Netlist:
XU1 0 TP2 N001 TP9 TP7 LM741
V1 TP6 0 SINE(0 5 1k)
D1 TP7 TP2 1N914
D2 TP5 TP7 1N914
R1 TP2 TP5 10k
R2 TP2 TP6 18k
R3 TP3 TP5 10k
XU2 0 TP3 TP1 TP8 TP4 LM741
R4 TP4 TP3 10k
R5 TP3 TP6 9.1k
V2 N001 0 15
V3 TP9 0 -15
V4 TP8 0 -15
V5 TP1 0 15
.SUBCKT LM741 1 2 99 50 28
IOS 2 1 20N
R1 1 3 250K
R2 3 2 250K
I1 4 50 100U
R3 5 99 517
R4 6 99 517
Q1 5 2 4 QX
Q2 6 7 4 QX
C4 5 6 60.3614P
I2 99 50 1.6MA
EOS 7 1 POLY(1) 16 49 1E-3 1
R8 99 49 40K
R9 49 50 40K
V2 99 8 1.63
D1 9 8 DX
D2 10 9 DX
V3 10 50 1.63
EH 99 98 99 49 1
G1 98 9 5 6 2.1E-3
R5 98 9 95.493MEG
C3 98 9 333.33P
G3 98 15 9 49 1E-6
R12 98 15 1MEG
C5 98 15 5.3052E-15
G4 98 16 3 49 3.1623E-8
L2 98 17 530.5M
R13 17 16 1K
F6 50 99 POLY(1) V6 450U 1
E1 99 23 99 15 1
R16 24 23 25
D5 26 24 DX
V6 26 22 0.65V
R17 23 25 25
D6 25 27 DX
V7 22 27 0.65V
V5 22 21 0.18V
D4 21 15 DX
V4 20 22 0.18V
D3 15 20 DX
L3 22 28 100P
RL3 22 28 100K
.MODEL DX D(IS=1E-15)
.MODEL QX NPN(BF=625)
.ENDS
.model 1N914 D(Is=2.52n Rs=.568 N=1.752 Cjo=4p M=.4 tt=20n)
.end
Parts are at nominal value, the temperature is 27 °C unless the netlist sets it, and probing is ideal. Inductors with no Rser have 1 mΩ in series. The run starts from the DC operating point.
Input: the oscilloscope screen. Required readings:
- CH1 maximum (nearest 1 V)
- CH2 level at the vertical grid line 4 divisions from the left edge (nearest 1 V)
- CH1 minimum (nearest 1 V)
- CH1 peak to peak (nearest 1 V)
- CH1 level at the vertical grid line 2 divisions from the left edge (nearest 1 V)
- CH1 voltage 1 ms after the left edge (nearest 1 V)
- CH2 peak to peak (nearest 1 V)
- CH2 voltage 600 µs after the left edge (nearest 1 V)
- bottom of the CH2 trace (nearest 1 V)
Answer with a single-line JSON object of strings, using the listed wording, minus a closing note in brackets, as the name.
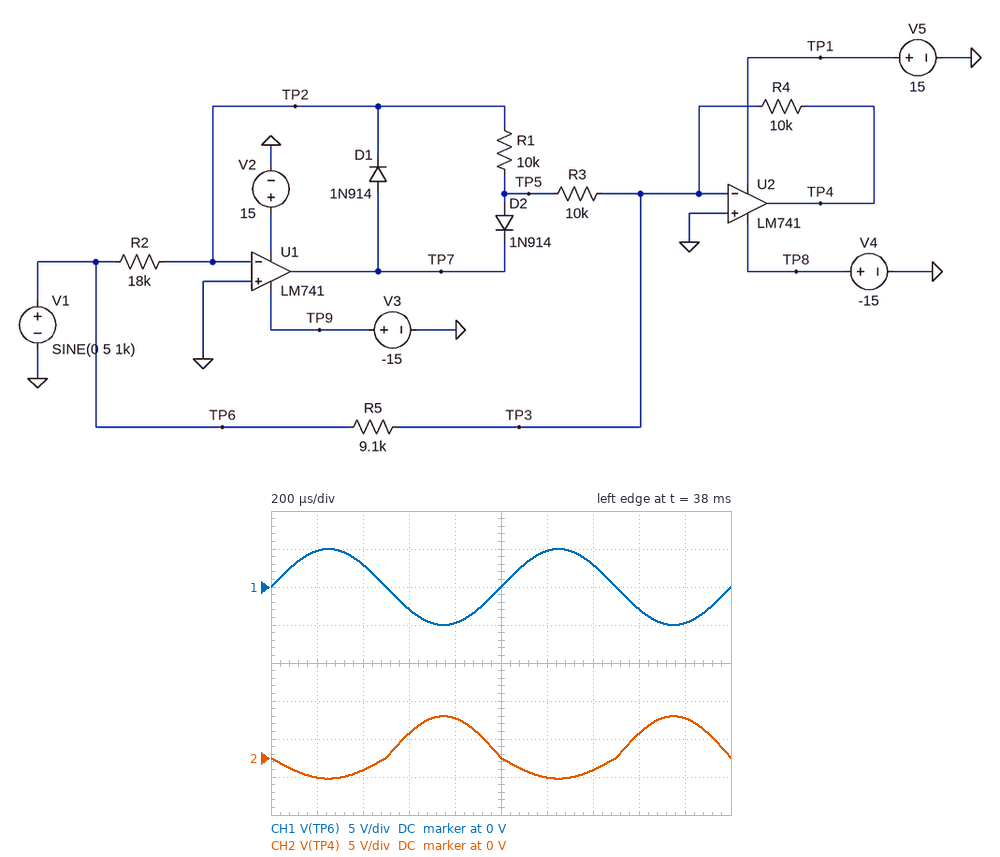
{"CH1 maximum": "5 V", "CH2 level at the vertical grid line 4 divisions from the left edge": "5 V", "CH1 minimum": "-5 V", "CH1 peak to peak": "10 V", "CH1 level at the vertical grid line 2 divisions from the left edge": "3 V", "CH1 voltage 1 ms after the left edge": "0 V", "CH2 peak to peak": "8 V", "CH2 voltage 600 µs after the left edge": "3 V", "bottom of the CH2 trace": "-3 V"}
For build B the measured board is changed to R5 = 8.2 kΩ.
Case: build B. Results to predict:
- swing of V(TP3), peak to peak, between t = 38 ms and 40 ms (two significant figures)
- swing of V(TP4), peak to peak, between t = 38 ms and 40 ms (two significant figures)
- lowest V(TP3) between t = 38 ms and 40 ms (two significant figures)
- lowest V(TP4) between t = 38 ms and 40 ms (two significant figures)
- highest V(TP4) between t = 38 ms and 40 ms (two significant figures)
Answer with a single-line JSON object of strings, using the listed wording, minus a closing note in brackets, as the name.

{"swing of V(TP3), peak to peak, between t = 38 ms and 40 ms": "14 mV", "swing of V(TP4), peak to peak, between t = 38 ms and 40 ms": "9.4 V", "lowest V(TP3) between t = 38 ms and 40 ms": "-6.1 mV", "lowest V(TP4) between t = 38 ms and 40 ms": "-3.3 V", "highest V(TP4) between t = 38 ms and 40 ms": "6.1 V"}
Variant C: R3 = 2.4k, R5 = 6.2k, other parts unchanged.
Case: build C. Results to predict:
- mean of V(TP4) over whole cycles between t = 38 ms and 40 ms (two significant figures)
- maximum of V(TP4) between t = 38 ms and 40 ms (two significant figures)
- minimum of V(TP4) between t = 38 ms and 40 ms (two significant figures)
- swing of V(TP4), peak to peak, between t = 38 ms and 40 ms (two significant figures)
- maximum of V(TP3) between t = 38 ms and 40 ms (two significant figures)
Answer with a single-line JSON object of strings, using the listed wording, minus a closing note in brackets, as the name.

{"mean of V(TP4) over whole cycles between t = 38 ms and 40 ms": "3.7 V", "maximum of V(TP4) between t = 38 ms and 40 ms": "8.1 V", "minimum of V(TP4) between t = 38 ms and 40 ms": "-200 mV", "swing of V(TP4), peak to peak, between t = 38 ms and 40 ms": "8.3 V", "maximum of V(TP3) between t = 38 ms and 40 ms": "10 mV"}
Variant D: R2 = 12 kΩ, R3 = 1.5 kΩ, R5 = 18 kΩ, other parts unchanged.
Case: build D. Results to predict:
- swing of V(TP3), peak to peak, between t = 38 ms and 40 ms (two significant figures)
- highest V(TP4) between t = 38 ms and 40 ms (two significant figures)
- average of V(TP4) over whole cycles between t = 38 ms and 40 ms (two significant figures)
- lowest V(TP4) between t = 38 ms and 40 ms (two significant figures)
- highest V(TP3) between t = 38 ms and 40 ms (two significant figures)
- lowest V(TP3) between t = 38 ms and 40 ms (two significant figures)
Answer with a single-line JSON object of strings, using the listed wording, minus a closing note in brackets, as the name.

{"swing of V(TP3), peak to peak, between t = 38 ms and 40 ms": "1.4 V", "highest V(TP4) between t = 38 ms and 40 ms": "14 V", "average of V(TP4) over whole cycles between t = 38 ms and 40 ms": "6.6 V", "lowest V(TP4) between t = 38 ms and 40 ms": "-89 mV", "highest V(TP3) between t = 38 ms and 40 ms": "28 mV", "lowest V(TP3) between t = 38 ms and 40 ms": "-1.3 V"}
